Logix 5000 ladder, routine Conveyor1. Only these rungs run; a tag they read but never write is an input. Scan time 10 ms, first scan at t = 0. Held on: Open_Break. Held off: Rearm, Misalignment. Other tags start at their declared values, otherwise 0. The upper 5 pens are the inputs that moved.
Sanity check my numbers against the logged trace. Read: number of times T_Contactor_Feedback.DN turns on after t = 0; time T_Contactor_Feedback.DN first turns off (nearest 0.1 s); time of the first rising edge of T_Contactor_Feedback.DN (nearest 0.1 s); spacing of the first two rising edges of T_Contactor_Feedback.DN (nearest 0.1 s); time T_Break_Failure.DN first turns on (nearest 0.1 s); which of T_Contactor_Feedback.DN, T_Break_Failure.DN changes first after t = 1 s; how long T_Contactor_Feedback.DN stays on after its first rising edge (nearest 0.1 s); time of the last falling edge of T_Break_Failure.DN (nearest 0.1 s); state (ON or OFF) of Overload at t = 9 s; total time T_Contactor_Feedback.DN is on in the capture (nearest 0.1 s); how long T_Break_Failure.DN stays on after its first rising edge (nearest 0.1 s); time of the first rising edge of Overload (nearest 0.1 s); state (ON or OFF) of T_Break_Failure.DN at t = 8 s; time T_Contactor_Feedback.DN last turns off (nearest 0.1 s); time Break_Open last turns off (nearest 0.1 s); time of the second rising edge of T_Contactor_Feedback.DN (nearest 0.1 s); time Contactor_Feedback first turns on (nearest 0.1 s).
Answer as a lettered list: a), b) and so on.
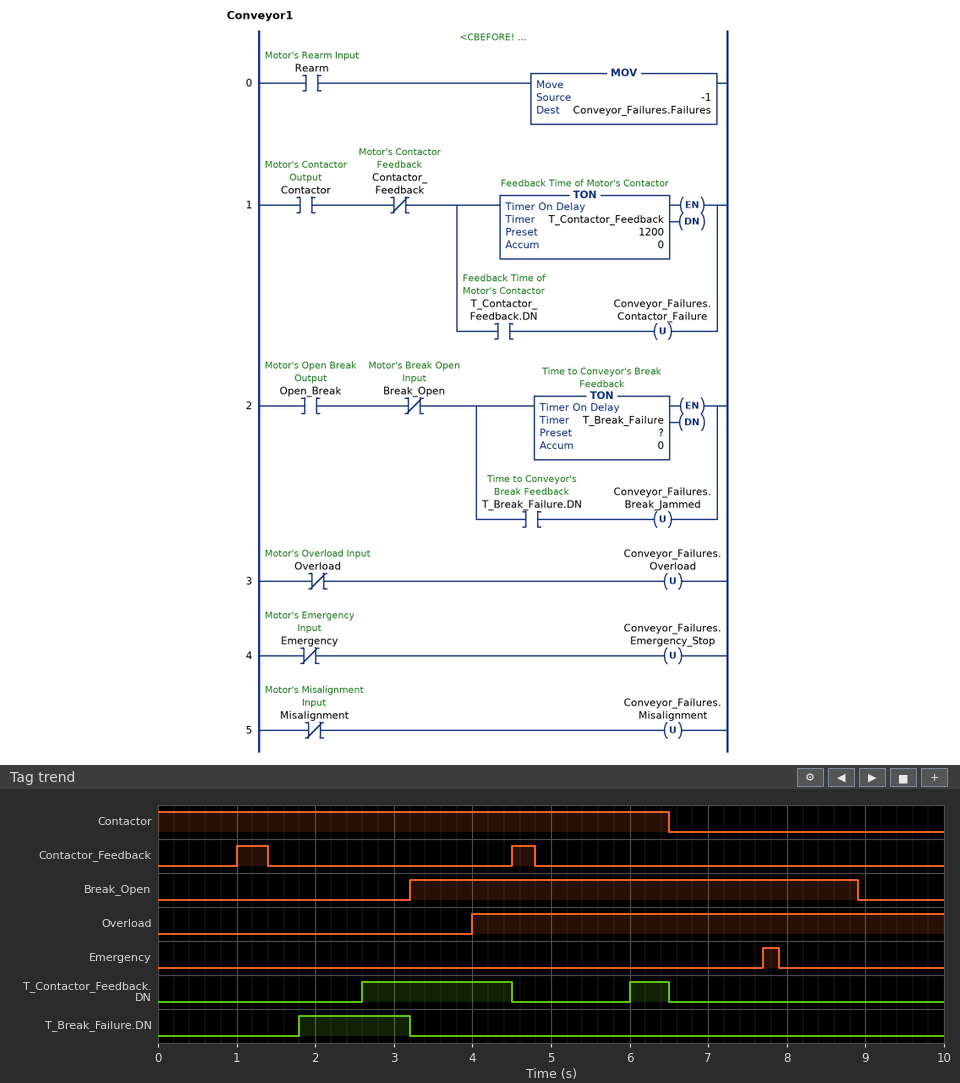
a) 2
b) 4.5 s
c) 2.6 s
d) 3.4 s
e) 1.8 s
f) T_Break_Failure.DN
g) 1.9 s
h) 3.2 s
i) ON
j) 2.4 s
k) 1.4 s
l) 4.0 s
m) OFF
n) 6.5 s
o) 8.9 s
p) 6.0 s
q) 1.0 s
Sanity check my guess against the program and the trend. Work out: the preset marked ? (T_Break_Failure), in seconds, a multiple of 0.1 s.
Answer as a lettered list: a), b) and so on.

a) 1.8 s
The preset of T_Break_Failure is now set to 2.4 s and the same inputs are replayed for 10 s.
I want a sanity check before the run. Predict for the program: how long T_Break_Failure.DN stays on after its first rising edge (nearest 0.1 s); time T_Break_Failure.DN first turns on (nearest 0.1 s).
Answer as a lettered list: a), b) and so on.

a) 0.8 s
b) 2.4 s
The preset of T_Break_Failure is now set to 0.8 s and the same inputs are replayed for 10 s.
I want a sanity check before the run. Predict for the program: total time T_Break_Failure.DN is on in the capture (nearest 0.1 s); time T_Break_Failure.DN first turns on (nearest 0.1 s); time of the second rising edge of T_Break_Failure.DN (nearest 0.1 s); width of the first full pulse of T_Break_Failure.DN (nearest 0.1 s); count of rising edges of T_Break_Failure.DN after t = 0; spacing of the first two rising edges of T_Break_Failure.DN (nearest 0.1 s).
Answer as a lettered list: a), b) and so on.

a) 2.7 s
b) 0.8 s
c) 9.7 s
d) 2.4 s
e) 2
f) 8.9 s
